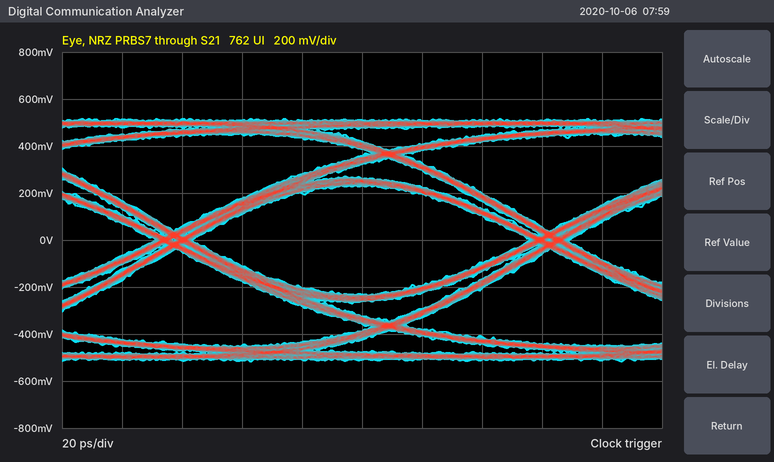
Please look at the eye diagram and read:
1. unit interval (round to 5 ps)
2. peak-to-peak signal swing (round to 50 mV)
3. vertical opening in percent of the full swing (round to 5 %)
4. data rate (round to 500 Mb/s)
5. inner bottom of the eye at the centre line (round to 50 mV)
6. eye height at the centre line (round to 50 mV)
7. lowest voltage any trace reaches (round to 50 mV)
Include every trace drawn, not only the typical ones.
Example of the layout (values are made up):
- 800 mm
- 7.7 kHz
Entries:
- 125 ps
- 1.05 V
- 45 %
- 8.0 Gb/s
- -250 mV
- 450 mV
- -500 mV
